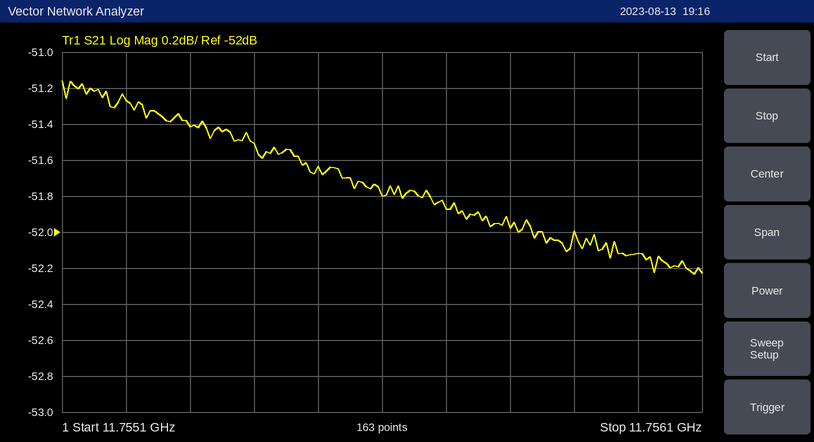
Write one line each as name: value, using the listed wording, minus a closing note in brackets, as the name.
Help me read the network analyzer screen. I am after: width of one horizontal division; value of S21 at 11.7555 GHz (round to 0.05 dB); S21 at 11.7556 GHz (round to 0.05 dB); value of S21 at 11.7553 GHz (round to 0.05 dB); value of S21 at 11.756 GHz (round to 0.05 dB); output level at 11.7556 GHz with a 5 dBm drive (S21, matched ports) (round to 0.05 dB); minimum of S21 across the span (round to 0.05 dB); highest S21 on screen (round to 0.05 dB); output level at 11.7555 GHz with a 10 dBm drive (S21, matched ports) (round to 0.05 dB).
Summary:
width of one horizontal division: 100 kHz
value of S21 at 11.7555 GHz: -51.65 dB
S21 at 11.7556 GHz: -51.80 dB
value of S21 at 11.7553 GHz: -51.40 dB
value of S21 at 11.756 GHz: -52.10 dB
output level at 11.7556 GHz with a 5 dBm drive (S21, matched ports): -46.80 dBm
minimum of S21 across the span: -52.25 dB
highest S21 on screen: -51.15 dB
output level at 11.7555 GHz with a 10 dBm drive (S21, matched ports): -41.65 dBm
